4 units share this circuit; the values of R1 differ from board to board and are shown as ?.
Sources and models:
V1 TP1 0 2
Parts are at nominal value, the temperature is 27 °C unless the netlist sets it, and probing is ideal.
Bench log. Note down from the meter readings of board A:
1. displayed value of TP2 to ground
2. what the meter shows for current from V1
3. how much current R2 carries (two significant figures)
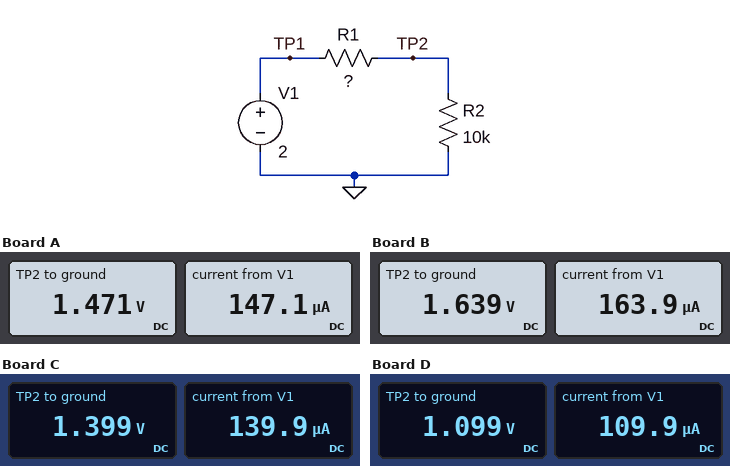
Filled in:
1.471 V
147.1 µA
150 µA
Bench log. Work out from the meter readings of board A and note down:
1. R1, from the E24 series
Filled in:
3.6 kΩ
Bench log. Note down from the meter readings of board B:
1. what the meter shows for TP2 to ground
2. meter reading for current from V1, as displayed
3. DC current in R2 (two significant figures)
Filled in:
1.639 V
163.9 µA
160 µA
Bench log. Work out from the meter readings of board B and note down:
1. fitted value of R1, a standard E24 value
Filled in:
2.2 kΩ
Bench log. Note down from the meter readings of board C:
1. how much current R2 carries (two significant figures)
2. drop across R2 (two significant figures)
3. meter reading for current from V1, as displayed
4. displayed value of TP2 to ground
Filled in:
140 µA
1.4 V
139.9 µA
1.399 V
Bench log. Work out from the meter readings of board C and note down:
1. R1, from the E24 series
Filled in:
4.3 kΩ
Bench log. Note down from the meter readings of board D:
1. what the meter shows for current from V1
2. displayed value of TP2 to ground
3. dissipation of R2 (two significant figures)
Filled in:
109.9 µA
1.099 V
120 µW
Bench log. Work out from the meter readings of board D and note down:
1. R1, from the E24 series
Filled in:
8.2 kΩ
